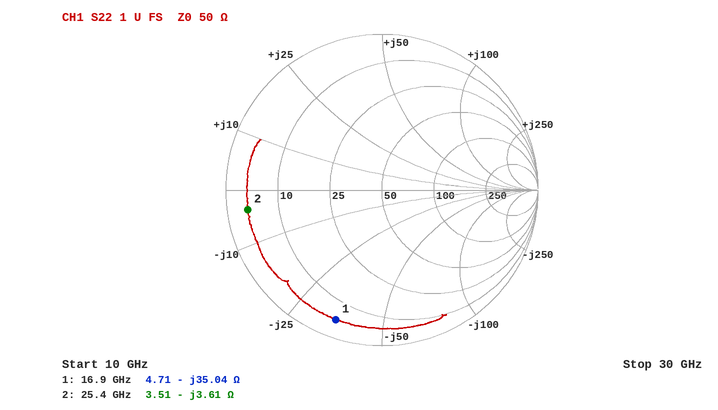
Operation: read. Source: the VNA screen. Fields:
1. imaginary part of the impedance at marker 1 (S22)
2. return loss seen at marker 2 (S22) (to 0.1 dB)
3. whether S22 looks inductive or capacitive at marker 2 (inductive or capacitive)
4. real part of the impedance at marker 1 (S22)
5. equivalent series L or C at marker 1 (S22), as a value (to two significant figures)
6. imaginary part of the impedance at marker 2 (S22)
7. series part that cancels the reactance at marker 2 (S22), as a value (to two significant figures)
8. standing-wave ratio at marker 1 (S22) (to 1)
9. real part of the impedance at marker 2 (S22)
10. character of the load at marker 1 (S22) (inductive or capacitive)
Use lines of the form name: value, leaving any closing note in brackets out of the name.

imaginary part of the impedance at marker 1: -35.04 Ω
return loss seen at marker 2 (S22): 1.2 dB
whether S22 looks inductive or capacitive at marker 2: capacitive
real part of the impedance at marker 1: 4.71 Ω
equivalent series L or C at marker 1 (S22), as a value: 270 fF
imaginary part of the impedance at marker 2: -3.61 Ω
series part that cancels the reactance at marker 2 (S22), as a value: 23 pH
standing-wave ratio at marker 1 (S22): 16
real part of the impedance at marker 2: 3.51 Ω
character of the load at marker 1 (S22): capacitive
